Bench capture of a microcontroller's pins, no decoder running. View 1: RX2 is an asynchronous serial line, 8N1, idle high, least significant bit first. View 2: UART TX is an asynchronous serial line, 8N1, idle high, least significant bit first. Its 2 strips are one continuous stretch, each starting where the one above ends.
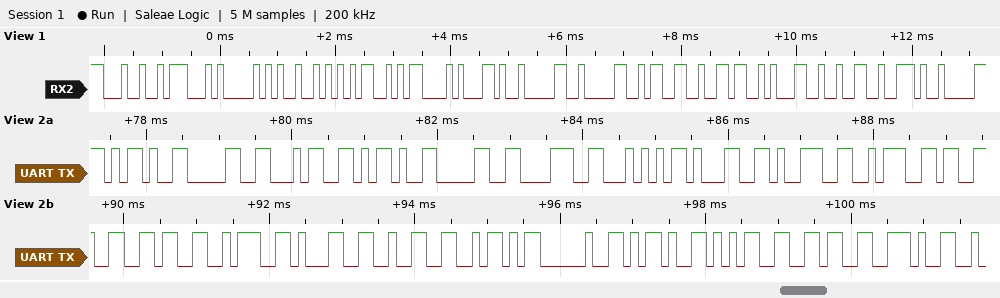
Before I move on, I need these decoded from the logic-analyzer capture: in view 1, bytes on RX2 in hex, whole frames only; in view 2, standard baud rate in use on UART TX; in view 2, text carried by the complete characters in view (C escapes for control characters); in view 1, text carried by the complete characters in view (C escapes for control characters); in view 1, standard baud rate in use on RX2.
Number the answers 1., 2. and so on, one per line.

1. 24 47 50 52 4D 43 2C 30 30 33 36 31 32 2E
2. 9600 baud
3. "-04-08T19:36:12Z -56."
4. "$GPRMC,003612."
5. 9600 baud
